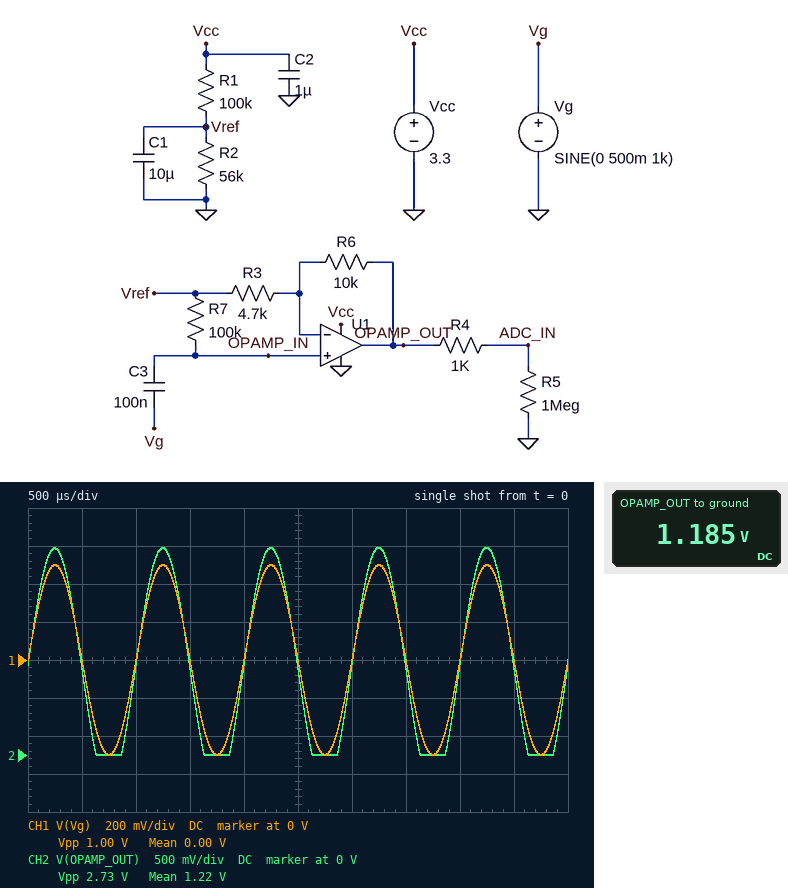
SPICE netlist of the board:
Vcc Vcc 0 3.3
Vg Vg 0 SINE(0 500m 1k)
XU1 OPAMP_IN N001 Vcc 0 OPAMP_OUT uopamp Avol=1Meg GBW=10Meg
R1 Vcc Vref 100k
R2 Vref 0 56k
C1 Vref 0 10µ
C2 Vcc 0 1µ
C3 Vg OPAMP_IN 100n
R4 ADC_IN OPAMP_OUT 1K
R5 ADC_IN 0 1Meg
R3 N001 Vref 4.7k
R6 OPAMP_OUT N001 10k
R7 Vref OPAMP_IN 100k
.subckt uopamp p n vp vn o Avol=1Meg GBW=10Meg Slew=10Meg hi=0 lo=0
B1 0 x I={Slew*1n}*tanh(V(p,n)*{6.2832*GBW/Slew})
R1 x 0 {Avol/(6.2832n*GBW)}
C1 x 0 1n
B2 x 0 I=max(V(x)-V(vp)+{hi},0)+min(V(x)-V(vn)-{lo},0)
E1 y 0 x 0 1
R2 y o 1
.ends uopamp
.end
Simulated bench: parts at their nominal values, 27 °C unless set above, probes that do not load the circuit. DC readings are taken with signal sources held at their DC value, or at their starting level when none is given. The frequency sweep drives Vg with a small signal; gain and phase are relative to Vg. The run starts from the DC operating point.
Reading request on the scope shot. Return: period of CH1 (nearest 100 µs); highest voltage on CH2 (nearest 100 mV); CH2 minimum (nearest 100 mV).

1.0 ms
2.7 V
0 V
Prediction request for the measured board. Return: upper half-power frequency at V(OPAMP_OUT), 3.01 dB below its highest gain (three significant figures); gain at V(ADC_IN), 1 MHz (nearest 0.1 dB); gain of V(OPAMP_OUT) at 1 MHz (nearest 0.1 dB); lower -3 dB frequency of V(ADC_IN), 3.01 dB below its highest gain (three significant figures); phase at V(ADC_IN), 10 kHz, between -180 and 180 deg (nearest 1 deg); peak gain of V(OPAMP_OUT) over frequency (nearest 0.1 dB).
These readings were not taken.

3.20 MHz
9.5 dB
9.5 dB
19.4 Hz
0 deg
9.9 dB
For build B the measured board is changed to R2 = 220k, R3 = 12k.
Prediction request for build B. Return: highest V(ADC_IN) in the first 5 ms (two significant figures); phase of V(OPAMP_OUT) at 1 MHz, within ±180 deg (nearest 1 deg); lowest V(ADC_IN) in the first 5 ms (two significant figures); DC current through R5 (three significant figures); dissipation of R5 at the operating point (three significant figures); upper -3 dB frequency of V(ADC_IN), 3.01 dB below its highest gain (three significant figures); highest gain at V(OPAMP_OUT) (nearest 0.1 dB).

3.2 V
-10 deg
1.3 V
2.27 µA
5.14 µW
5.45 MHz
5.3 dB
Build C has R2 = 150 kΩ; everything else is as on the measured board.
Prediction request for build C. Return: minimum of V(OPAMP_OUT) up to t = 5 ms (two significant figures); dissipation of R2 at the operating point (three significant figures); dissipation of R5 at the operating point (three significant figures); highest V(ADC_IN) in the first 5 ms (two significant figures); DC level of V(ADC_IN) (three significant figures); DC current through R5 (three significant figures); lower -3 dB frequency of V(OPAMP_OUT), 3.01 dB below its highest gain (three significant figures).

390 mV
26.1 µW
3.91 µW
3.3 V
1.98 V
1.98 µA
19.4 Hz
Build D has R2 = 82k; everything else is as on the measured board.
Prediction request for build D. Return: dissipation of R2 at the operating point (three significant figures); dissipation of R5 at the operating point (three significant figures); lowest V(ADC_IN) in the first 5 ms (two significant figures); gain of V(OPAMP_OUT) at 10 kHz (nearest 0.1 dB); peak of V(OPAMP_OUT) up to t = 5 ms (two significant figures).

27.0 µW
2.21 µW
-1.9 mV
9.9 dB
3.0 V
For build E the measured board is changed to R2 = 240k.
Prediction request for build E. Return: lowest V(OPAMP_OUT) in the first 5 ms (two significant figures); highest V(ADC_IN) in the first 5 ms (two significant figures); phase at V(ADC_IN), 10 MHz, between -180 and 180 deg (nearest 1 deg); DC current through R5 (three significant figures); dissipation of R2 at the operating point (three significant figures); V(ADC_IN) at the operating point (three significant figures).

740 mV
3.3 V
-72 deg
2.33 µA
22.6 µW
2.33 V
